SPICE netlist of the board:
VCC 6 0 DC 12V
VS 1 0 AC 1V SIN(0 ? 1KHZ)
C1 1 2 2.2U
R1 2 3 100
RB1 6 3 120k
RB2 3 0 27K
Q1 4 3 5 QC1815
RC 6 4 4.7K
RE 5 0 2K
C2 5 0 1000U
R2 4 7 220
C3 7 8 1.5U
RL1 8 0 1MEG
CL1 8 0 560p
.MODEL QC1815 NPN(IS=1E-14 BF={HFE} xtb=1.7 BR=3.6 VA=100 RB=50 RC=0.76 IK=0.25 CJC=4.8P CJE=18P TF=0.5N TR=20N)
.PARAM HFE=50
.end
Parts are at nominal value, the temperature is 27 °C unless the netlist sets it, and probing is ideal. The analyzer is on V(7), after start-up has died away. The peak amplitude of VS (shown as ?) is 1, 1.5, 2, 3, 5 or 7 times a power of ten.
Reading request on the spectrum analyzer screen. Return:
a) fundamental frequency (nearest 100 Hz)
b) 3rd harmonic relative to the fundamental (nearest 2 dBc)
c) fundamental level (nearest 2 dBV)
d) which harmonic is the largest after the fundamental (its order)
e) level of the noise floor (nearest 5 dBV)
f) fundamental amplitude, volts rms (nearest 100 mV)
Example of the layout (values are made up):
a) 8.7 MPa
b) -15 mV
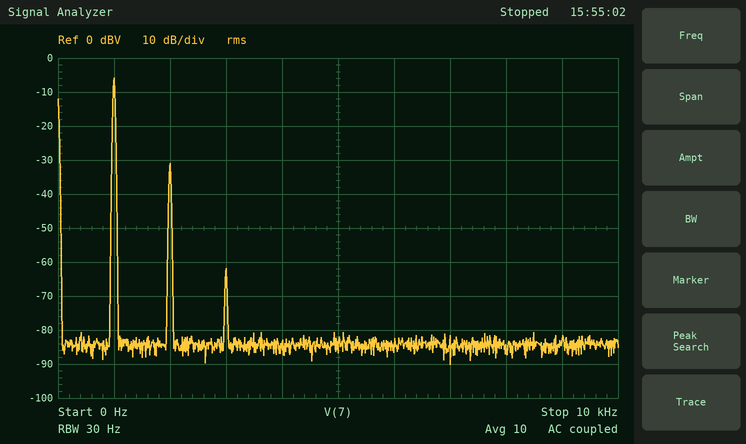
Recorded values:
a) 1.0 kHz
b) -56 dBc
c) -6 dBV
d) 2
e) -85 dBV
f) 500 mV
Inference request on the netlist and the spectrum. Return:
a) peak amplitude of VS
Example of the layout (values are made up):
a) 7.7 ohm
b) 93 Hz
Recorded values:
a) 7 mV
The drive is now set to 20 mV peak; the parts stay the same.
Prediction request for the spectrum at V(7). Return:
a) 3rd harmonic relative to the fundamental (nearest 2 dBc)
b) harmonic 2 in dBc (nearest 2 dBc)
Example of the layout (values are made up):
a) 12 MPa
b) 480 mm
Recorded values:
a) -38 dBc
b) -16 dBc
